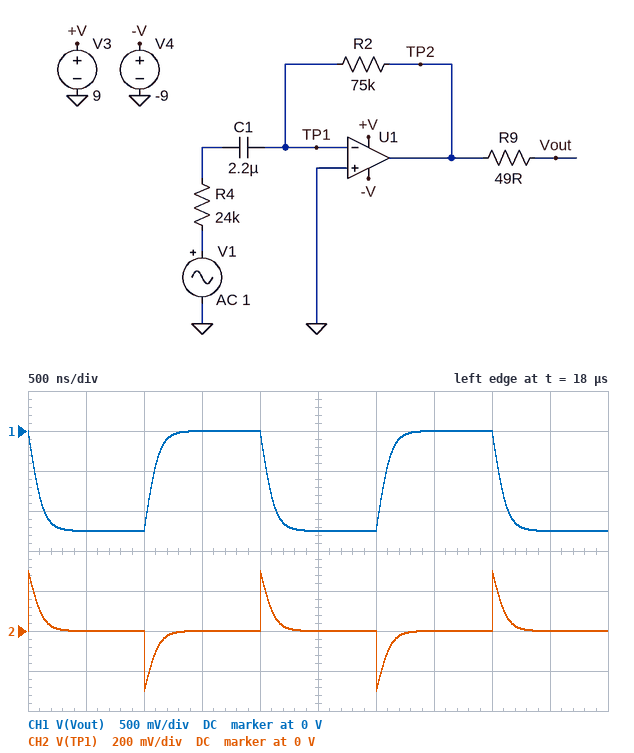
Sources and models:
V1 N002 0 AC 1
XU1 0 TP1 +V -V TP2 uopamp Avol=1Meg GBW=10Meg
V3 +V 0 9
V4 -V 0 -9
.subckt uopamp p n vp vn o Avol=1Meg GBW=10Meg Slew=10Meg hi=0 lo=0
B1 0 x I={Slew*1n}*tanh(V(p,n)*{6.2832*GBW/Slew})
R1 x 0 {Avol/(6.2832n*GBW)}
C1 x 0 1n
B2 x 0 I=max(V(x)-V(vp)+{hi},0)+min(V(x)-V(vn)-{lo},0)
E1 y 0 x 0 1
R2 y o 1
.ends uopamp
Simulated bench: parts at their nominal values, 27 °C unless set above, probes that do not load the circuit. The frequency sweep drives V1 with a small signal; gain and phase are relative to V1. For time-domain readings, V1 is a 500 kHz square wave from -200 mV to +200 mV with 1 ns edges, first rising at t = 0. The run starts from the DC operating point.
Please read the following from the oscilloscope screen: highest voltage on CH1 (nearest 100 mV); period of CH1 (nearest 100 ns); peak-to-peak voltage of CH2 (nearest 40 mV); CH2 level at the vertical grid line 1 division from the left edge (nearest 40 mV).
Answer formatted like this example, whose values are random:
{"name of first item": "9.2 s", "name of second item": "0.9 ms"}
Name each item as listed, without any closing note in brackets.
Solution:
{"highest voltage on CH1": "0 V", "period of CH1": "2.0 µs", "peak-to-peak voltage of CH2": "600 mV", "CH2 level at the vertical grid line 1 division from the left edge": "0 V"}
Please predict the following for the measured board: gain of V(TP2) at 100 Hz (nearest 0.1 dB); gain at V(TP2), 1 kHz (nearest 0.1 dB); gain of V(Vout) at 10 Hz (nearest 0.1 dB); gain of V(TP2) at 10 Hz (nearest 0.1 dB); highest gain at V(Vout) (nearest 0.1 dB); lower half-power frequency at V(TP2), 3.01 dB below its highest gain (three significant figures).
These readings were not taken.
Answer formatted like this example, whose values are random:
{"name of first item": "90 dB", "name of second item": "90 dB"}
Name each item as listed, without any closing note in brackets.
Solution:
{"gain of V(TP2) at 100 Hz": "9.9 dB", "gain at V(TP2), 1 kHz": "9.9 dB", "gain of V(Vout) at 10 Hz": "9.5 dB", "gain of V(TP2) at 10 Hz": "9.5 dB", "highest gain at V(Vout)": "9.9 dB", "lower half-power frequency at V(TP2), 3.01 dB below its highest gain": "3.01 Hz"}
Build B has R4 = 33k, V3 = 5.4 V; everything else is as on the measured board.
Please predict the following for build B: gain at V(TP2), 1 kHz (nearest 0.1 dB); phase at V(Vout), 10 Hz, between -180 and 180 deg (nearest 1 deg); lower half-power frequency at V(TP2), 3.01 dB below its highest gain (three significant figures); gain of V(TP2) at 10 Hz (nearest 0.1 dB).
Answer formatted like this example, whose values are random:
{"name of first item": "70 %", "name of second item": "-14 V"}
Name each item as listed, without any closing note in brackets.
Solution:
{"gain at V(TP2), 1 kHz": "7.1 dB", "phase at V(Vout), 10 Hz, between -180 and 180 deg": "-168 deg", "lower half-power frequency at V(TP2), 3.01 dB below its highest gain": "2.19 Hz", "gain of V(TP2) at 10 Hz": "6.9 dB"}
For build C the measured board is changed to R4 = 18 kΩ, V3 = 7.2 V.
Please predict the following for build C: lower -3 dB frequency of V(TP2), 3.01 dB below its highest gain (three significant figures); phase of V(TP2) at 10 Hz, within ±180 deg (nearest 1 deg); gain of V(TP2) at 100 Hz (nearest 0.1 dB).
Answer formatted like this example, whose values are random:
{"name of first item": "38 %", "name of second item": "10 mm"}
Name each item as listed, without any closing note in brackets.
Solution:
{"lower -3 dB frequency of V(TP2), 3.01 dB below its highest gain": "4.02 Hz", "phase of V(TP2) at 10 Hz, within ±180 deg": "-158 deg", "gain of V(TP2) at 100 Hz": "12.4 dB"}
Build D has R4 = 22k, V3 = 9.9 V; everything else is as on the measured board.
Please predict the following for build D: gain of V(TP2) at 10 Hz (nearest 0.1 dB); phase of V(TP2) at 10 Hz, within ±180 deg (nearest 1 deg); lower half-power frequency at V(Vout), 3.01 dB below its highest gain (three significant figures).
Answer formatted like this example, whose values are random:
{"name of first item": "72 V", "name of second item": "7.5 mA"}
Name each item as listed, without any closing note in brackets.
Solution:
{"gain of V(TP2) at 10 Hz": "10.2 dB", "phase of V(TP2) at 10 Hz, within ±180 deg": "-162 deg", "lower half-power frequency at V(Vout), 3.01 dB below its highest gain": "3.29 Hz"}
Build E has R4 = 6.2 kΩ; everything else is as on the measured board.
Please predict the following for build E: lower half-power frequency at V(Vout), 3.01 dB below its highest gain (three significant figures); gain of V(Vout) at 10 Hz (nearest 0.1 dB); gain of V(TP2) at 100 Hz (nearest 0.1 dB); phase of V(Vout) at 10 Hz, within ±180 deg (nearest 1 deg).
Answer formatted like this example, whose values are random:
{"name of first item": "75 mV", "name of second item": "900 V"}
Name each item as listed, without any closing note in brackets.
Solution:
{"lower half-power frequency at V(Vout), 3.01 dB below its highest gain": "11.7 Hz", "gain of V(Vout) at 10 Hz": "17.9 dB", "gain of V(TP2) at 100 Hz": "21.6 dB", "phase of V(Vout) at 10 Hz, within ±180 deg": "-131 deg"}
